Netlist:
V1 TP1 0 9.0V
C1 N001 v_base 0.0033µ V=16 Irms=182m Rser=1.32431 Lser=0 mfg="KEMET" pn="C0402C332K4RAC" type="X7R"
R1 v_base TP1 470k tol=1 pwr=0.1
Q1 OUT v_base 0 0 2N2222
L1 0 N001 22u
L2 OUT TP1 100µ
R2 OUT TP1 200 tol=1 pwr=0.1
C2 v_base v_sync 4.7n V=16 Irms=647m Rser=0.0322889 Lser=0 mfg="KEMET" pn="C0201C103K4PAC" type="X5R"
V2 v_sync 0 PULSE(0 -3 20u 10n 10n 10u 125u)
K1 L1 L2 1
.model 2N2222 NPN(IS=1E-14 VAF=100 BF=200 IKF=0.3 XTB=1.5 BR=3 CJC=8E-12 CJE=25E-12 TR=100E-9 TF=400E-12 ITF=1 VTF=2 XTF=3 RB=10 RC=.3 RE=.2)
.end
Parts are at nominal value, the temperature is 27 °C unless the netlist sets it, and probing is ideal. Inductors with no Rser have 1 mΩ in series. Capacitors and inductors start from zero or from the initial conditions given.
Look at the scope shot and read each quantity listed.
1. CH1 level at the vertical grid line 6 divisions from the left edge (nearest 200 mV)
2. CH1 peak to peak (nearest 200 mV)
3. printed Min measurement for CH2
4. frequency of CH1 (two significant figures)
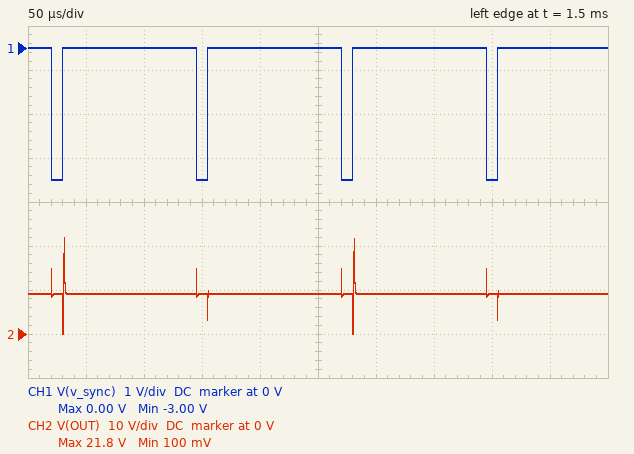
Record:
0 V
3.0 V
100 mV
8.0 kHz
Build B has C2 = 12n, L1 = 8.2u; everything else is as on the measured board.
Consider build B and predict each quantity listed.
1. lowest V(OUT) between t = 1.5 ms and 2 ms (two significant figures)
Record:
83 mV
